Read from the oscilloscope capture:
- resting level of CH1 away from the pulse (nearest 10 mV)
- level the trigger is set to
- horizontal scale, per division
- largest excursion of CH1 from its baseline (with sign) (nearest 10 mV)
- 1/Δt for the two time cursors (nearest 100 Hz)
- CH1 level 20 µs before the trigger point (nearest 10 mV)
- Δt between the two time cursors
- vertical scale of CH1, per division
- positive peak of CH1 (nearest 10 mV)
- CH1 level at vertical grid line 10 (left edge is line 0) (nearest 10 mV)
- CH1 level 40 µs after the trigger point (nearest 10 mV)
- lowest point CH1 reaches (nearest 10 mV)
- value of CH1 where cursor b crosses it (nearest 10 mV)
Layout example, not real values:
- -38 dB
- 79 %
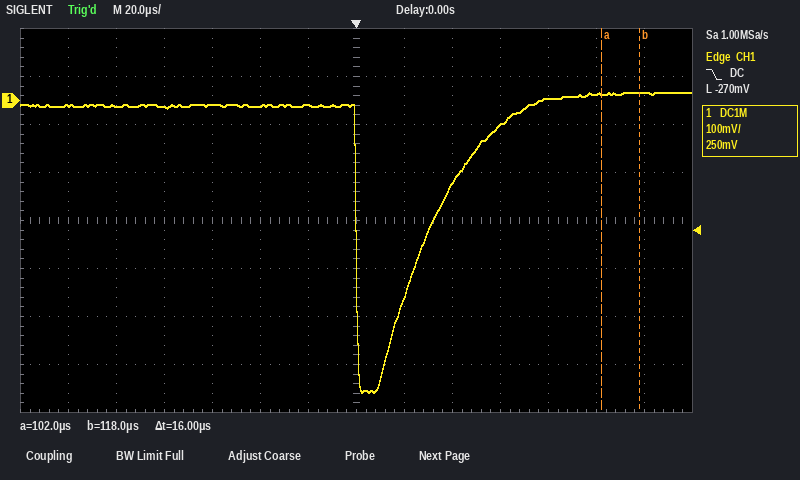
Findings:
- -10 mV
- -270 mV
- 20 µs
- -600 mV
- 62.5 kHz
- -10 mV
- 16 µs
- 100 mV
- 20 mV
- -50 mV
- -170 mV
- -610 mV
- 20 mV
